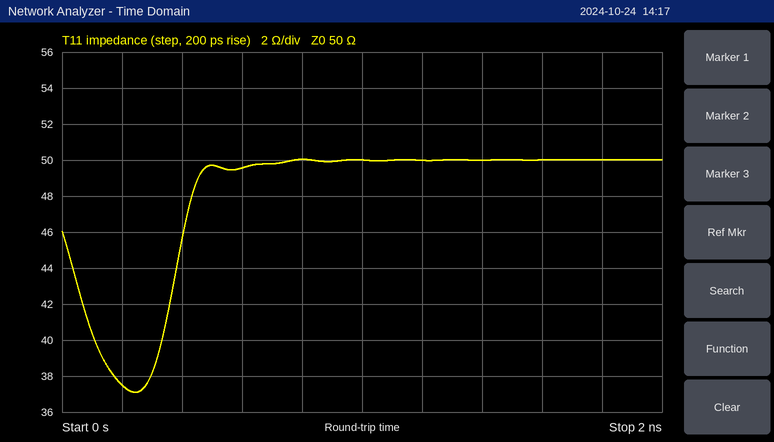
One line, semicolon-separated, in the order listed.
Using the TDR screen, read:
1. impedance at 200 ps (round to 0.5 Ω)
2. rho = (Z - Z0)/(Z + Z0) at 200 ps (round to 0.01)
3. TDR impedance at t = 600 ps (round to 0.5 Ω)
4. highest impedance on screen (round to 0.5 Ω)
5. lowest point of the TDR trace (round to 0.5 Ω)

37.5 Ω; -0.14; 49.5 Ω; 50.0 Ω; 37.0 Ω
